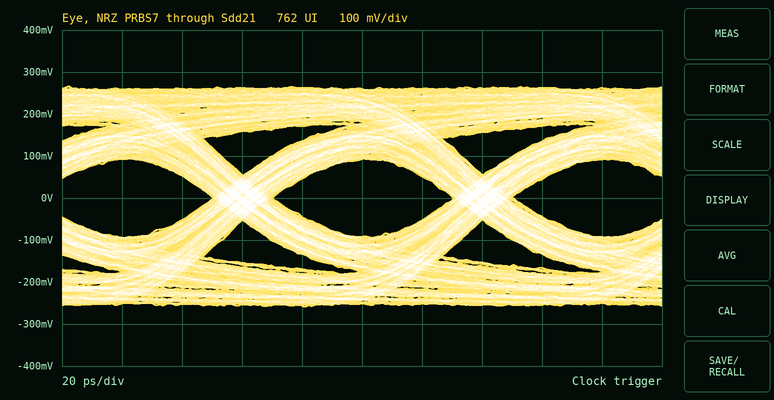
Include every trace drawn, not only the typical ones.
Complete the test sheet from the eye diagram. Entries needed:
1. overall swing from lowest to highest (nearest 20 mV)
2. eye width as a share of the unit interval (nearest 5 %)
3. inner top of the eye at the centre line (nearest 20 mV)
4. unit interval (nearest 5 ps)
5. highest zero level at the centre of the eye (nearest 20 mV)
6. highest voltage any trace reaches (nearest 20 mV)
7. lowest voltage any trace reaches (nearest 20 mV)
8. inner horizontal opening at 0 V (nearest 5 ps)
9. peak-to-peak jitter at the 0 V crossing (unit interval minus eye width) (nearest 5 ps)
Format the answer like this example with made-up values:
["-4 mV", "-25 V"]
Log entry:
["520 mV", "75 %", "100 mV", "80 ps", "-100 mV", "260 mV", "-260 mV", "60 ps", "20 ps"]
